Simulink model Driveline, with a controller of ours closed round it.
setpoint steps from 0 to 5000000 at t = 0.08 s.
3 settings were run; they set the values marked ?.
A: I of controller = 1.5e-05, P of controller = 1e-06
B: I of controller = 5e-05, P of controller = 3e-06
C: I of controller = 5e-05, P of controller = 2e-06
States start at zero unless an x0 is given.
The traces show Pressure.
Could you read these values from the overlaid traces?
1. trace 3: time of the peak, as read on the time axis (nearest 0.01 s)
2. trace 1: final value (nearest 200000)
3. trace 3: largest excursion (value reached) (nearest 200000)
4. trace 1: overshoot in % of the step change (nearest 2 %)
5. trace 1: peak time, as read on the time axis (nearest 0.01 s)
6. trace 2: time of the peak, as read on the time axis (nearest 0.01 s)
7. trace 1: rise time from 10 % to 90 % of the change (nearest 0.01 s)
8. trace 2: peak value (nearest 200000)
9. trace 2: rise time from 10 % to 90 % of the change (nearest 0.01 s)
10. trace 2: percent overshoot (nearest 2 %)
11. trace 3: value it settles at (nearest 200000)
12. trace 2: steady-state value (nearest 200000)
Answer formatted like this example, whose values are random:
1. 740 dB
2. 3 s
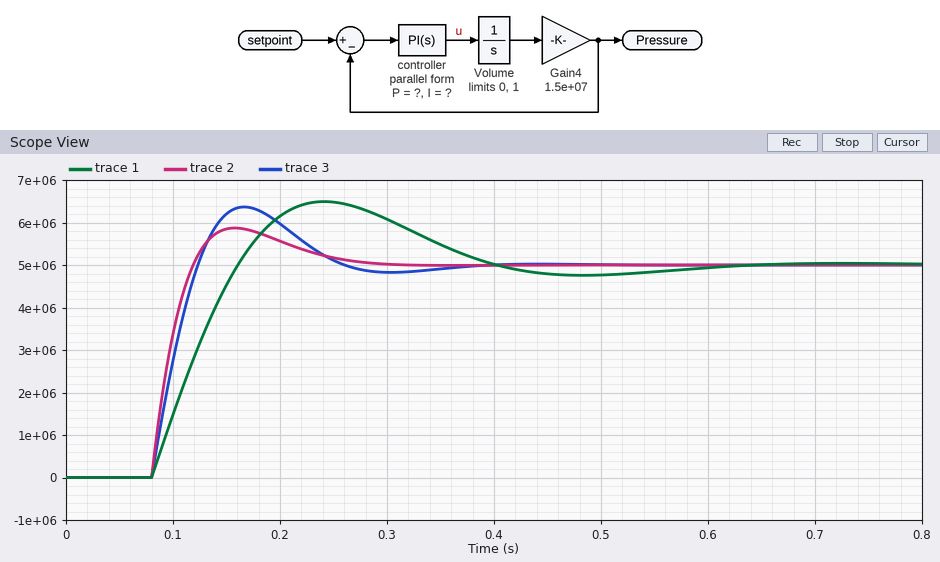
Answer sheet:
1. 0.17 s
2. 5000000
3. 6400000
4. 30 %
5. 0.24 s
6. 0.16 s
7. 0.06 s
8. 5800000
9. 0.03 s
10. 18 %
11. 5000000
12. 5000000
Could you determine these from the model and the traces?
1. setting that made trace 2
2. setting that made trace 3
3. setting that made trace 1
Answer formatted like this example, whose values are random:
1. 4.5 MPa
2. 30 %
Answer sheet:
1. B
2. C
3. A
